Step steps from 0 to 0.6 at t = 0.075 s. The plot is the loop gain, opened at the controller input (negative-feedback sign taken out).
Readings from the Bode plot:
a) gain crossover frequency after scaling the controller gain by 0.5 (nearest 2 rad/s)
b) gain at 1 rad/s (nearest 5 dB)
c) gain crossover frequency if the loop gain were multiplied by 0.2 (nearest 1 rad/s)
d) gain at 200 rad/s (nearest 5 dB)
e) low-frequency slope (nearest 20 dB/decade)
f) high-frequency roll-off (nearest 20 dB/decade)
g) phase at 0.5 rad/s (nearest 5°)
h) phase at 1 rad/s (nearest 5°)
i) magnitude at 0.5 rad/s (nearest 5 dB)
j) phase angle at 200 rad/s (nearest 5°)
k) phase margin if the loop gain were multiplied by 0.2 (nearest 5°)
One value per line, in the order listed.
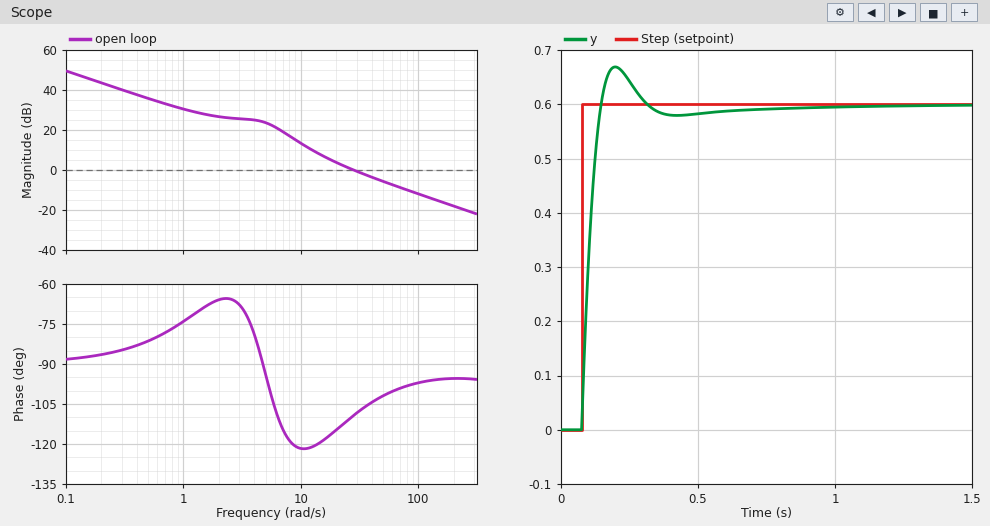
16 rad/s
30 dB
10 rad/s
-20 dB
-20 dB/decade
-20 dB/decade
-80°
-75°
35 dB
-95°
60°
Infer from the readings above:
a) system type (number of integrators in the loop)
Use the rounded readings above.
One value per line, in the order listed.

1
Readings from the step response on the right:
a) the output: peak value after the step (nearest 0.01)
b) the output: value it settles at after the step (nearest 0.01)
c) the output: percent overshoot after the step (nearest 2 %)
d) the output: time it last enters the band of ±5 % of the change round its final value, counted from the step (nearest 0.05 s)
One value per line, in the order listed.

0.67
0.60
12 %
0.20 s
